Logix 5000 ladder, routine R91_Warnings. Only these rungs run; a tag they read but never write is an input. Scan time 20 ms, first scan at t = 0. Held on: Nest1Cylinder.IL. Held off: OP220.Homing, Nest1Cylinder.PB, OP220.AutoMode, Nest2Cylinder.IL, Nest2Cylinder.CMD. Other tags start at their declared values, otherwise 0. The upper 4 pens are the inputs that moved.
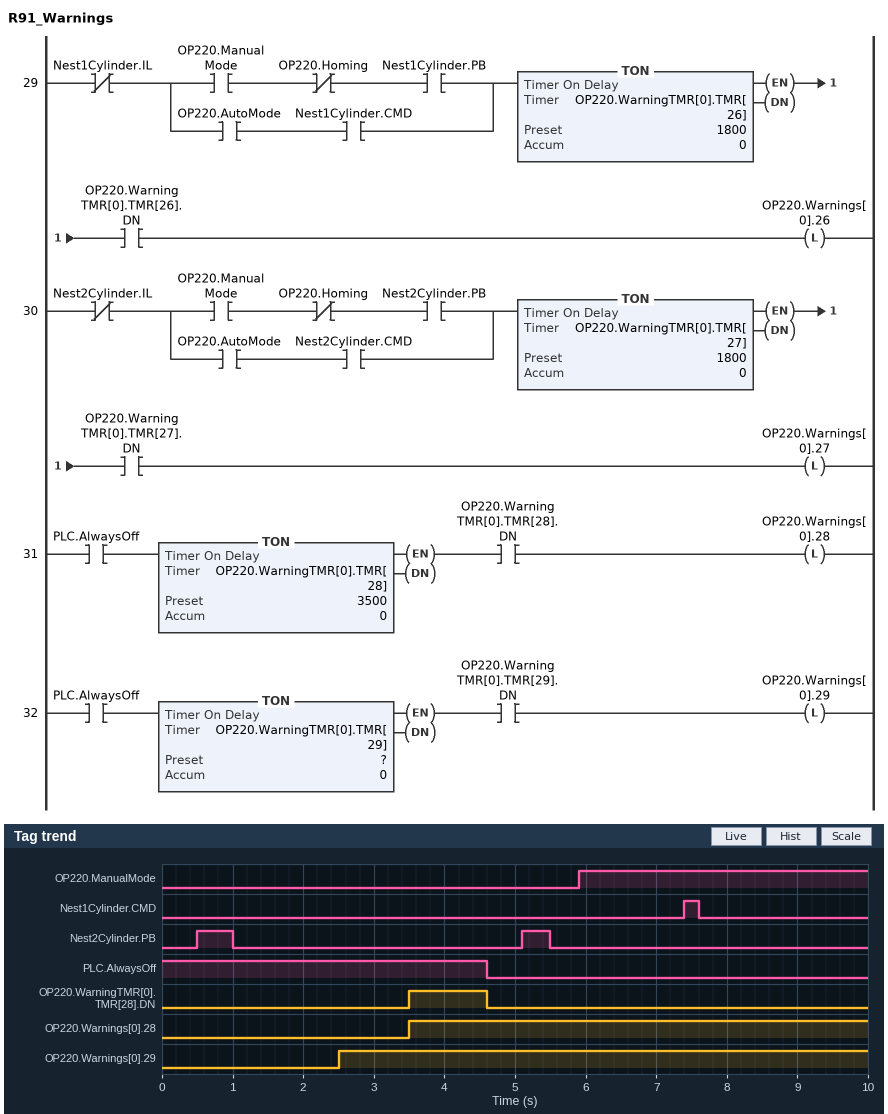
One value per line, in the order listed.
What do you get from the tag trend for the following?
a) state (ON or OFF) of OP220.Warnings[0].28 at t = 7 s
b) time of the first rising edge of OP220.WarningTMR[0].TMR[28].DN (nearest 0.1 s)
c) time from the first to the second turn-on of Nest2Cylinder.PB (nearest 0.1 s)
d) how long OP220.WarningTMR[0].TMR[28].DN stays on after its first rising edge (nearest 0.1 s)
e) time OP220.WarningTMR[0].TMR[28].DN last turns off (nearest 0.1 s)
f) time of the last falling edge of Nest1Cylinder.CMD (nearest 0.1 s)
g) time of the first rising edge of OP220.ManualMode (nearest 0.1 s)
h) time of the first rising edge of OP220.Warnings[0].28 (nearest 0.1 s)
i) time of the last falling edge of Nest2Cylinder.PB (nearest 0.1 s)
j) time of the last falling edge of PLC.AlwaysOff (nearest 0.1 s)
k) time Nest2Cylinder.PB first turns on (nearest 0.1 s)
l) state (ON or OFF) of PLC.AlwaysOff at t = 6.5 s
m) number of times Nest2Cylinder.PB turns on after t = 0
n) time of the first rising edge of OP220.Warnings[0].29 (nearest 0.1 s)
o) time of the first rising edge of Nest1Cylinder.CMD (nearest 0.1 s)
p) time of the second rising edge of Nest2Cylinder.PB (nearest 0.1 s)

ON
3.5 s
4.6 s
1.1 s
4.6 s
7.6 s
5.9 s
3.5 s
5.5 s
4.6 s
0.5 s
OFF
2
2.5 s
7.4 s
5.1 s
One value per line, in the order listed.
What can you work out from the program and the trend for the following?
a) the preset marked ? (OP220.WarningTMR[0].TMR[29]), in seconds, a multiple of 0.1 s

2.5 s
